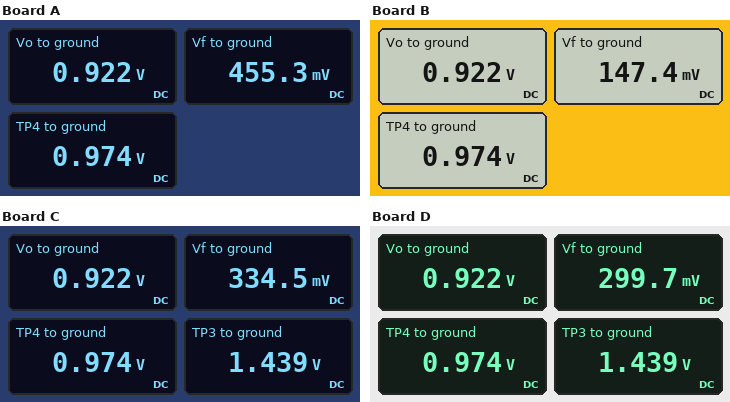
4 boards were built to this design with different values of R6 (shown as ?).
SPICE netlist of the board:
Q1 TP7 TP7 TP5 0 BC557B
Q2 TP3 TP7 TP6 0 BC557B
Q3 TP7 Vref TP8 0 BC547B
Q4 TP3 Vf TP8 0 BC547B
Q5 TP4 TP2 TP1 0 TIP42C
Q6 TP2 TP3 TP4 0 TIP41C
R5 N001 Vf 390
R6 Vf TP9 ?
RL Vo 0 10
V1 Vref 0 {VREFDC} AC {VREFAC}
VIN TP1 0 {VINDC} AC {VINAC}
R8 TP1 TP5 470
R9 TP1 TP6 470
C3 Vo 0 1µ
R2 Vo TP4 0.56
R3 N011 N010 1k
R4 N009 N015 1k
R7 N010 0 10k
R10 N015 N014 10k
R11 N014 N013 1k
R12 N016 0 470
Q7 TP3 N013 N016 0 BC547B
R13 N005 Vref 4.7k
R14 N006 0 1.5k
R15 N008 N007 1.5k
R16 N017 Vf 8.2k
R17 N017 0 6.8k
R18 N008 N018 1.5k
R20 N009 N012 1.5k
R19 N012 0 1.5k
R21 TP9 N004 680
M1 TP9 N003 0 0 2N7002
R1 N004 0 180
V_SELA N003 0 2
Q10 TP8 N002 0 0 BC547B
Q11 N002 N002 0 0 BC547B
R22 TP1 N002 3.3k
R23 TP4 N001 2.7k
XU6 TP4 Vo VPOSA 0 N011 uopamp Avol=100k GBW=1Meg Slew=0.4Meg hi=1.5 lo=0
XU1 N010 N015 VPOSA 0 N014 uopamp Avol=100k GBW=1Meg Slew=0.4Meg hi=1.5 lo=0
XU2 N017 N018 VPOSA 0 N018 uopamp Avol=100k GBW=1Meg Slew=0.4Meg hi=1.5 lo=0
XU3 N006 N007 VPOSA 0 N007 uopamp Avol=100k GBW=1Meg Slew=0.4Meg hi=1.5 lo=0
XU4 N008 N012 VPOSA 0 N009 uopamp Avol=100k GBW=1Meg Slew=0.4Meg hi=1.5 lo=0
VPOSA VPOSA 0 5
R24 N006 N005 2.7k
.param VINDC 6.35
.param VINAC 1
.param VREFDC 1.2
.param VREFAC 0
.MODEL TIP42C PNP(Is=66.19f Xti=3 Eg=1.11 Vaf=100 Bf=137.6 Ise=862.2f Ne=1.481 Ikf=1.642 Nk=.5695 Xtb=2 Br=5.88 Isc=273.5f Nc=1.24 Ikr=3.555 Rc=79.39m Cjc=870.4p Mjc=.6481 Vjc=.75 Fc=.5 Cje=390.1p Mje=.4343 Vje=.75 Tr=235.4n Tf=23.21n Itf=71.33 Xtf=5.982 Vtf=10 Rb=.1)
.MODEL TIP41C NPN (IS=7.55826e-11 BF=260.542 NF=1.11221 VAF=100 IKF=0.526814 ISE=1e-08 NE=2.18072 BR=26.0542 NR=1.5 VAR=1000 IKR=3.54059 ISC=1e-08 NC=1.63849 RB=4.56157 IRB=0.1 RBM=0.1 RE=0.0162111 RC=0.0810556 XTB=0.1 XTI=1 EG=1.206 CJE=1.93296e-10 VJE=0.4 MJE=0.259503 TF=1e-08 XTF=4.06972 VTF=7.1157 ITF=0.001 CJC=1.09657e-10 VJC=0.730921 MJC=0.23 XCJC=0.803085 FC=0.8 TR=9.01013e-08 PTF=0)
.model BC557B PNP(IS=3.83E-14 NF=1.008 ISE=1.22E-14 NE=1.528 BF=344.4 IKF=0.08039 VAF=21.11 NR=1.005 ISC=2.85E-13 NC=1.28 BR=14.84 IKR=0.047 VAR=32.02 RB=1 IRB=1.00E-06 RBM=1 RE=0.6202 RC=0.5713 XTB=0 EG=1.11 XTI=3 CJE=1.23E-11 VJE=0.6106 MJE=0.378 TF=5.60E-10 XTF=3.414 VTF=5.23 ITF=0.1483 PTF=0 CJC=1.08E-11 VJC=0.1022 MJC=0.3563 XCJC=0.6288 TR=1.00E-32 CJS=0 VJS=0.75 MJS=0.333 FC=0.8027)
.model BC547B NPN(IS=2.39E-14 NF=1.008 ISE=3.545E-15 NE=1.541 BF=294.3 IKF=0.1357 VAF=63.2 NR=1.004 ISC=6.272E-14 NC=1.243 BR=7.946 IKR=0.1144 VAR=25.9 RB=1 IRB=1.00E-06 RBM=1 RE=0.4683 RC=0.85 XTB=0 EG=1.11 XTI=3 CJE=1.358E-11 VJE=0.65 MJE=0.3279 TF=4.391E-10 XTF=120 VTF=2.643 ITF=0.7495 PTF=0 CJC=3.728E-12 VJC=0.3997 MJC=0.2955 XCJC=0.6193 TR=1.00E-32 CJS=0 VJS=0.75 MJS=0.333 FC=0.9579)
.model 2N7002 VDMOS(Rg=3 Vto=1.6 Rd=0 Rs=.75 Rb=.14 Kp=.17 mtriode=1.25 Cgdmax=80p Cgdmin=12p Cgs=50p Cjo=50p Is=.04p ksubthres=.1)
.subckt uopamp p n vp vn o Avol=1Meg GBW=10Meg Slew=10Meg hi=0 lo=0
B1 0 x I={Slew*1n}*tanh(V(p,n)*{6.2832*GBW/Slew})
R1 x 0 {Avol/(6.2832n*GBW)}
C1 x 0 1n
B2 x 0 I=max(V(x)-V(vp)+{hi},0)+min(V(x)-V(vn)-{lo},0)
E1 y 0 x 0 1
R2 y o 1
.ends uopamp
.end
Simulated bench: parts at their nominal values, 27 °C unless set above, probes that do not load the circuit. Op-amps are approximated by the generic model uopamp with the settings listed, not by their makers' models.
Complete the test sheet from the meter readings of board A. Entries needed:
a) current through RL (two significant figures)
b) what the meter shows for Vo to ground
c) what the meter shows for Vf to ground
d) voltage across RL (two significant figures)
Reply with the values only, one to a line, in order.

92 mA
0.922 V
455.3 mV
920 mV
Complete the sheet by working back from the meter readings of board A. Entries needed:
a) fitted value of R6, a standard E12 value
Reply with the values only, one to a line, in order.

3.3 kΩ
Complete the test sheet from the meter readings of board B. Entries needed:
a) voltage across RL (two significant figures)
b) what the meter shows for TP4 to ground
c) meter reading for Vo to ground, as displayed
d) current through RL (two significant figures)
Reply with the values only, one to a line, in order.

920 mV
0.974 V
0.922 V
92 mA
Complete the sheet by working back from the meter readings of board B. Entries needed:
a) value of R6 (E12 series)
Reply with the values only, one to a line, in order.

560 Ω
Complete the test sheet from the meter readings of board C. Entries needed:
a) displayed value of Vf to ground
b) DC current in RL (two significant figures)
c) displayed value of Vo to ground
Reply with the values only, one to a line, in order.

334.5 mV
92 mA
0.922 V
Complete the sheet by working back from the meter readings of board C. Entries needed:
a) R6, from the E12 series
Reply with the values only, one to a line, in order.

1.8 kΩ
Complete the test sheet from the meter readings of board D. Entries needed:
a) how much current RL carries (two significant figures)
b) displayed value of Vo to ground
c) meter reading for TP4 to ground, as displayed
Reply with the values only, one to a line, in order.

92 mA
0.922 V
0.974 V
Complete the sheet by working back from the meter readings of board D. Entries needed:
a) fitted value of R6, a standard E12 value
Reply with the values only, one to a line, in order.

1.5 kΩ
